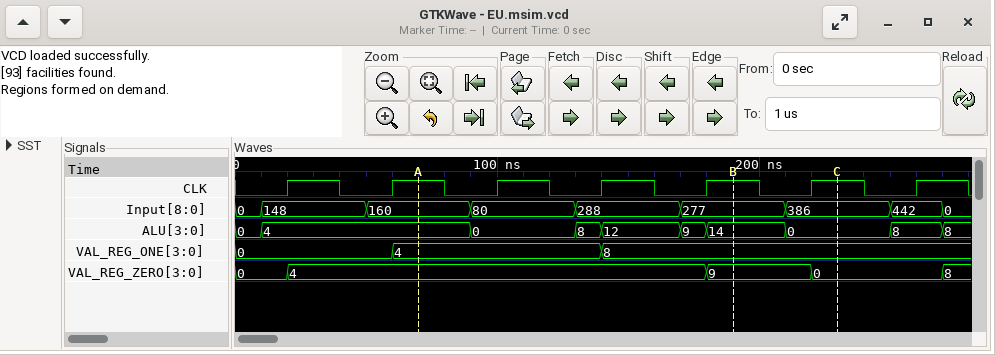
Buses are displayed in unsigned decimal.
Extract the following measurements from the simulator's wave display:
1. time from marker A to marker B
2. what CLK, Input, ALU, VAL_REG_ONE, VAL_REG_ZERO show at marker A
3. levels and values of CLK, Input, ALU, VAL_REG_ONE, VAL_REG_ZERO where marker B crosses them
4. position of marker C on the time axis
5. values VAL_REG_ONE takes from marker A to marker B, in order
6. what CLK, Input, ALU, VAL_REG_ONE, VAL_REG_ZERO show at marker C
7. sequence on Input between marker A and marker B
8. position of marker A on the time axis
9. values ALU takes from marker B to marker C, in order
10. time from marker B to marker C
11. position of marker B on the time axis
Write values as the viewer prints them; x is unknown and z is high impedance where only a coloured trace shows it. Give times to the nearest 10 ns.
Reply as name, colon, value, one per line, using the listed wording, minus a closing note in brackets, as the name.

time from marker A to marker B: 120 ns
what CLK, Input, ALU, VAL_REG_ONE, VAL_REG_ZERO show at marker A: CLK=1, Input=160, ALU=4, VAL_REG_ONE=4, VAL_REG_ZERO=4
levels and values of CLK, Input, ALU, VAL_REG_ONE, VAL_REG_ZERO where marker B crosses them: CLK=1, Input=277, ALU=14, VAL_REG_ONE=8, VAL_REG_ZERO=9
position of marker C on the time axis: 230 ns
values VAL_REG_ONE takes from marker A to marker B, in order: 4, 8
what CLK, Input, ALU, VAL_REG_ONE, VAL_REG_ZERO show at marker C: CLK=1, Input=386, ALU=0, VAL_REG_ONE=8, VAL_REG_ZERO=0
sequence on Input between marker A and marker B: 160, 80, 288, 277
position of marker A on the time axis: 70 ns
values ALU takes from marker B to marker C, in order: 14, 0
time from marker B to marker C: 40 ns
position of marker B on the time axis: 190 ns
